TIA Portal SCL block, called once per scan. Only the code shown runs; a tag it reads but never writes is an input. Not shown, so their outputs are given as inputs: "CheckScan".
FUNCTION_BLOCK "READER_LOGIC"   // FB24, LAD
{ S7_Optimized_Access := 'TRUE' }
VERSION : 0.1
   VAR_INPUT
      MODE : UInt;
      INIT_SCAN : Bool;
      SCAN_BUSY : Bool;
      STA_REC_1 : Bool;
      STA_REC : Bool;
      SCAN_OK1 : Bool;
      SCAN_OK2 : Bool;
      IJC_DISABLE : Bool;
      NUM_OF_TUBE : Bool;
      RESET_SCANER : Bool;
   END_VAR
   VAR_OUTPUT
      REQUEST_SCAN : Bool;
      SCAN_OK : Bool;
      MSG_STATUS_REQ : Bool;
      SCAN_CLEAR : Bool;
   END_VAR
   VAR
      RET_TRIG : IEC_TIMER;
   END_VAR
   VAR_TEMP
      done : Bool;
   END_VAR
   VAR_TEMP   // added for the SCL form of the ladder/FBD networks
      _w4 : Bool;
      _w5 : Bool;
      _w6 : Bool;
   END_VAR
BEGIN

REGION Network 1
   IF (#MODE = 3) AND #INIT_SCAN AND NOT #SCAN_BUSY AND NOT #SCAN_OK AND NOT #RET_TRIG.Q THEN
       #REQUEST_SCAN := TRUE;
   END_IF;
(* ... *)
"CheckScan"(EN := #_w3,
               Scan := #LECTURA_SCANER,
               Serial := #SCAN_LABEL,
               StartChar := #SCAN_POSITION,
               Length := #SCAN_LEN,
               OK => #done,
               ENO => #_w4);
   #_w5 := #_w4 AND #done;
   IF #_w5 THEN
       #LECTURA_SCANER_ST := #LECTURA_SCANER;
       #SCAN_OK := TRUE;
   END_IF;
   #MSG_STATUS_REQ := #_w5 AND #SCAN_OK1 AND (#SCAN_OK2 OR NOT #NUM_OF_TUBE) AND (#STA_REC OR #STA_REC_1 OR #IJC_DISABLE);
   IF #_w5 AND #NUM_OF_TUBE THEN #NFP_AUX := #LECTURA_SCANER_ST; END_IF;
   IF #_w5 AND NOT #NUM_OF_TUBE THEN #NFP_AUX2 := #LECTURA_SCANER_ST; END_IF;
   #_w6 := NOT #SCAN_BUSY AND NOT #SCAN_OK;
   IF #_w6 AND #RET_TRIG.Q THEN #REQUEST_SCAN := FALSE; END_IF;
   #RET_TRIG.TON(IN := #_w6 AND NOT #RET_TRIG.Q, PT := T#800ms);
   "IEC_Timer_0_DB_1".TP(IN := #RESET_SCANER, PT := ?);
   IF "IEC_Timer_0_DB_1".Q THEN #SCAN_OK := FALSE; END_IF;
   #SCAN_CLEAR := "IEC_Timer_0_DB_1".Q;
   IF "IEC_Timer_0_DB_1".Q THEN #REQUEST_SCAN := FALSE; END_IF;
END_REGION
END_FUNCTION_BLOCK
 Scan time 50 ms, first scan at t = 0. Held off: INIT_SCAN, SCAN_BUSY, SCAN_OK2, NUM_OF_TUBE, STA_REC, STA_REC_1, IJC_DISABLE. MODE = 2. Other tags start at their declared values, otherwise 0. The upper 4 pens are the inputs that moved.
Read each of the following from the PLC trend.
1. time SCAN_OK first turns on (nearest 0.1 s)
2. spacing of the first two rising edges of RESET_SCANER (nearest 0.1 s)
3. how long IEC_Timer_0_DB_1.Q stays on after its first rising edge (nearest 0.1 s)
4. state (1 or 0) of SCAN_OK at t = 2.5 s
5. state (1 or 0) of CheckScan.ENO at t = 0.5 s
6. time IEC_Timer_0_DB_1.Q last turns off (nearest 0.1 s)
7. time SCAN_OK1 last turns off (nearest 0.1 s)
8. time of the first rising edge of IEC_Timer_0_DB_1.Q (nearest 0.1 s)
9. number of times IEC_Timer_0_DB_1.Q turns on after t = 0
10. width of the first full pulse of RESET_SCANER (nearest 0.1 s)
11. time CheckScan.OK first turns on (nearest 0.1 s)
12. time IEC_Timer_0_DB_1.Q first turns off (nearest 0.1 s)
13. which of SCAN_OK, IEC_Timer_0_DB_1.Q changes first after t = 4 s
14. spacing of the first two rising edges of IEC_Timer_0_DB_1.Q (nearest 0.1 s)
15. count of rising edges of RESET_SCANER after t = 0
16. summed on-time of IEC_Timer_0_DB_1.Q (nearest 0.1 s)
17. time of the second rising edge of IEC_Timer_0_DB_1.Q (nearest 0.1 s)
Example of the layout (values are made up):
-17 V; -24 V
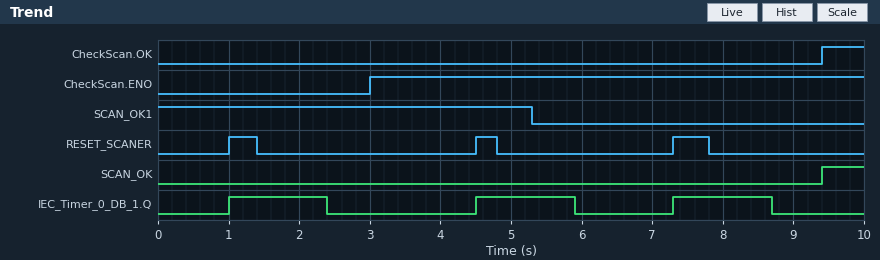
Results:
9.4 s; 3.5 s; 1.4 s; 0; 0; 8.7 s; 5.3 s; 1.0 s; 3; 0.4 s; 9.4 s; 2.4 s; IEC_Timer_0_DB_1.Q; 3.5 s; 3; 4.2 s; 4.5 s
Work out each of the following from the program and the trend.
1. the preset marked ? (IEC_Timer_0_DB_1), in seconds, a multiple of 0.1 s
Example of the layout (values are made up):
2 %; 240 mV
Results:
1.4 s
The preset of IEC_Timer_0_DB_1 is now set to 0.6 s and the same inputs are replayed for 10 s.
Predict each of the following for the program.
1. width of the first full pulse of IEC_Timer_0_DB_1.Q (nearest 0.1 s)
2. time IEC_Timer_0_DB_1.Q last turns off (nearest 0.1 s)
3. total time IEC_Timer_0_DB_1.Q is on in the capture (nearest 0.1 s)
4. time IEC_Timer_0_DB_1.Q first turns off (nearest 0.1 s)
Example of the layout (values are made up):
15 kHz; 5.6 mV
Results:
0.6 s; 7.9 s; 1.8 s; 1.6 s
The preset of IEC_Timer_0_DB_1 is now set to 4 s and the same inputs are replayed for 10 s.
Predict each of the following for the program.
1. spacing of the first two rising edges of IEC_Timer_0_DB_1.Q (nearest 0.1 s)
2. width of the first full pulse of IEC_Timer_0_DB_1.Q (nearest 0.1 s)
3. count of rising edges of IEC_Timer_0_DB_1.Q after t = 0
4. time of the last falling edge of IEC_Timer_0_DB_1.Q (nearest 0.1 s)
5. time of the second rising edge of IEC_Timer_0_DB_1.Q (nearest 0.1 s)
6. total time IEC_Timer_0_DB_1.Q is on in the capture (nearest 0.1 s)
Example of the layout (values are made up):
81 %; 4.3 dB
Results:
6.3 s; 4.0 s; 2; 5.0 s; 7.3 s; 6.7 s
